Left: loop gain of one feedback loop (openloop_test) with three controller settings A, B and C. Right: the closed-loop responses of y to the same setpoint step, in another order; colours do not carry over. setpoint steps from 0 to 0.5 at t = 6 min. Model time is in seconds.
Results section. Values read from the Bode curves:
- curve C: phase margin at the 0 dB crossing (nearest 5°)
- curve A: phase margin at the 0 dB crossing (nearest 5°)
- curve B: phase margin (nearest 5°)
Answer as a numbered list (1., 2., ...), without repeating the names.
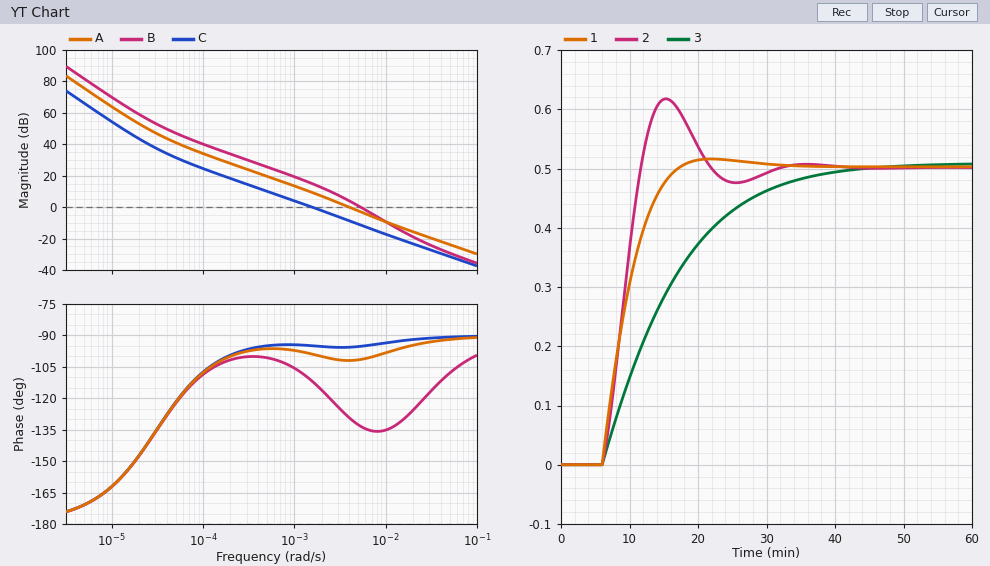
1. 85°
2. 80°
3. 45°
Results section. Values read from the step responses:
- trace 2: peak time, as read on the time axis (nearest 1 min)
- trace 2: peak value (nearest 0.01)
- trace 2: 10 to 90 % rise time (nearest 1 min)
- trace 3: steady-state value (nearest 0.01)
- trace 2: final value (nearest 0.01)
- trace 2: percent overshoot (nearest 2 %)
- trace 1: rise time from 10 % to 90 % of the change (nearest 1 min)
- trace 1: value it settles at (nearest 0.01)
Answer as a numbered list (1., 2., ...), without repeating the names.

1. 15 min
2. 0.62
3. 4 min
4. 0.51
5. 0.50
6. 24 %
7. 7 min
8. 0.50
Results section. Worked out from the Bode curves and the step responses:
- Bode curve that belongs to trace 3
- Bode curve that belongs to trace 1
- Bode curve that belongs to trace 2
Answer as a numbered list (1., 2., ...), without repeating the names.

1. C
2. A
3. B
